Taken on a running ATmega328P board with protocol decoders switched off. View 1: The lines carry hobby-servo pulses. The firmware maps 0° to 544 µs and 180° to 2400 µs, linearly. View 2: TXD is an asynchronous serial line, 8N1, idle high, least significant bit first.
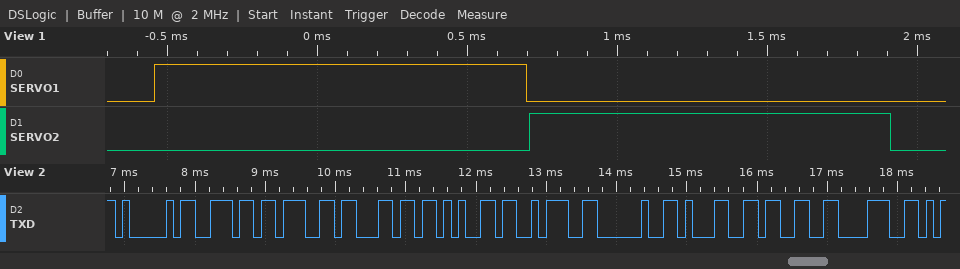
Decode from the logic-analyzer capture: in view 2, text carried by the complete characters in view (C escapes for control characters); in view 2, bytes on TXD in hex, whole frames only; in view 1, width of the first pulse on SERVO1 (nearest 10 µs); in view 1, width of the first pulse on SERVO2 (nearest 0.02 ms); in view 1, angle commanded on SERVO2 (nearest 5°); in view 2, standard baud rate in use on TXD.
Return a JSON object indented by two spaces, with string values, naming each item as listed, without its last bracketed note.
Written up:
{
  "in view 2, text carried by the complete characters in view": "\"Angle: 138\"",
  "in view 2, bytes on TXD in hex, whole frames only": "41 6E 67 6C 65 3A 20 31 33 38",
  "in view 1, width of the first pulse on SERVO1": "1240 µs",
  "in view 1, width of the first pulse on SERVO2": "1.20 ms",
  "in view 1, angle commanded on SERVO2": "65°",
  "in view 2, standard baud rate in use on TXD": "9600 baud"
}
